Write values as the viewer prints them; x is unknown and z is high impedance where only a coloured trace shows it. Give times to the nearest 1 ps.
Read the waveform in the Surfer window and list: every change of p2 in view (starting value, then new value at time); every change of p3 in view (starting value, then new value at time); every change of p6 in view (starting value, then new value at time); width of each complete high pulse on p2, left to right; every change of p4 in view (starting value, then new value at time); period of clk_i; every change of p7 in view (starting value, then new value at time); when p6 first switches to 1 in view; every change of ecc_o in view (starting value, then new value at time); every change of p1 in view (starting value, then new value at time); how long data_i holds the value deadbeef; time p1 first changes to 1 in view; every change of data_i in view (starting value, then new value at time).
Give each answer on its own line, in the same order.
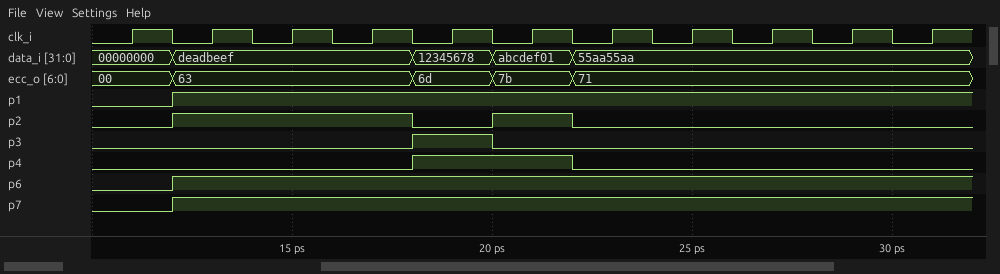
0, 1 at 12 ps, 0 at 18 ps, 1 at 20 ps, 0 at 22 ps
0, 1 at 18 ps, 0 at 20 ps
0, 1 at 12 ps
6 ps, 2 ps
0, 1 at 18 ps, 0 at 22 ps
2 ps
0, 1 at 12 ps
12 ps
00, 63 at 12 ps, 6d at 18 ps, 7b at 20 ps, 71 at 22 ps
0, 1 at 12 ps
6 ps
12 ps
00000000, deadbeef at 12 ps, 12345678 at 18 ps, abcdef01 at 20 ps, 55aa55aa at 22 ps
